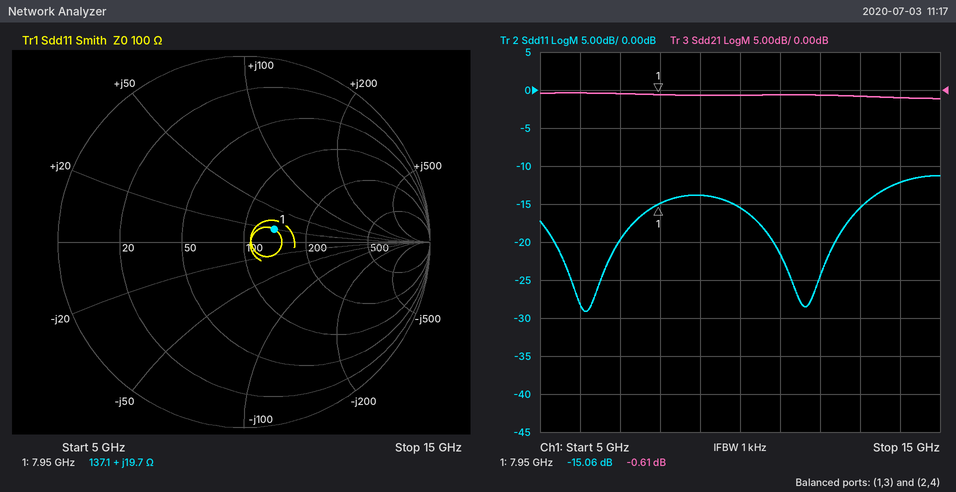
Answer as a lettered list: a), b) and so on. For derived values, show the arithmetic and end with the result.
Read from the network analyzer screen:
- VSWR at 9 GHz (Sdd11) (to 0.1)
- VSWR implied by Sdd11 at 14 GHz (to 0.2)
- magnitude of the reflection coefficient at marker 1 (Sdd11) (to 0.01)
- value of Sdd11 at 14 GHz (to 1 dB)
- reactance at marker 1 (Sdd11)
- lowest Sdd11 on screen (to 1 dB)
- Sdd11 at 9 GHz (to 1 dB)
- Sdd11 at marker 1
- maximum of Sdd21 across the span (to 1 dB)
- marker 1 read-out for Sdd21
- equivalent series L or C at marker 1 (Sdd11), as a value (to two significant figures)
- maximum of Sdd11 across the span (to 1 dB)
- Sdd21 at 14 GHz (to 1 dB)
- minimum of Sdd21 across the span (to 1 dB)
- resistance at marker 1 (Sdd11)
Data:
a) |Γ| = 10^(-14/20) = 0.1995; VSWR = (1 + 0.1995)/(1 − 0.1995) ≈ 1.5
b) |Γ| = 10^(-12/20) = 0.2512; VSWR = (1 + 0.2512)/(1 − 0.2512) ≈ 1.67, so 1.6 to the nearest 0.2
c) 10^(-15.06/20) ≈ 0.18
d) -12 dB
e) +19.7 Ω
f) -29 dB
g) -14 dB
h) -15.06 dB
i) 0 dB
j) -0.61 dB
k) L = 19.7 Ω/(2π × 7.95 GHz) ≈ 394 pH, so 390 pH to two significant figures
l) -11 dB
m) -1 dB
n) -1 dB
o) 137.1 Ω
